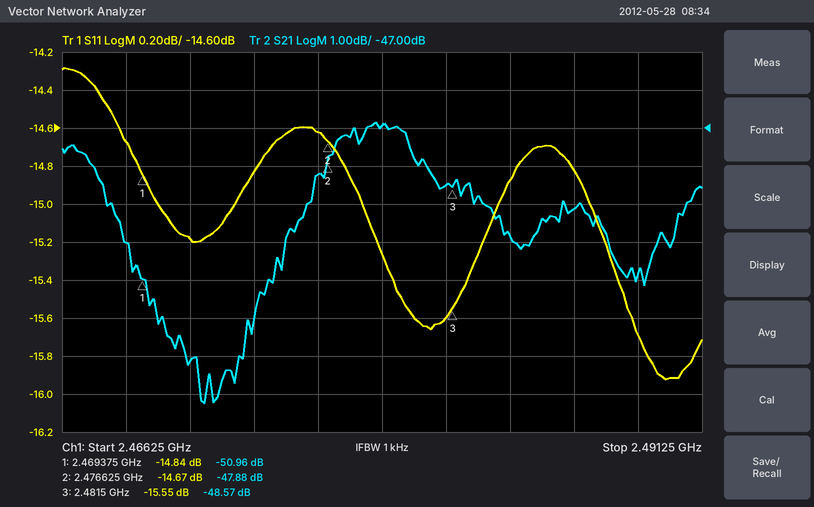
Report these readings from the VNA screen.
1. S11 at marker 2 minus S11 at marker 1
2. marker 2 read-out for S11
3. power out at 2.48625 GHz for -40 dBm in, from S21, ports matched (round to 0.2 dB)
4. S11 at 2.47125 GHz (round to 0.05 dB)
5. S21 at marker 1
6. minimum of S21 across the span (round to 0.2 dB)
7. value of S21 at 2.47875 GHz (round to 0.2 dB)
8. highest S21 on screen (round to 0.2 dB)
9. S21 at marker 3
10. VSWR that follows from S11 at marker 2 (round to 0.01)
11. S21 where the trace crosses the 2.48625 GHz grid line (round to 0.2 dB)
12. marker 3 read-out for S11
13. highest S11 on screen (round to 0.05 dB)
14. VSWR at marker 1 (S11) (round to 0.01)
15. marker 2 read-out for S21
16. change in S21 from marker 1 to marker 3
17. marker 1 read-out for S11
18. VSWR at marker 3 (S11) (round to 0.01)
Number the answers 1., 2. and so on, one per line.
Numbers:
1. 0.17 dB
2. -14.67 dB
3. -89.2 dBm
4. -15.20 dB
5. -50.96 dB
6. -54.2 dB
7. -47.0 dB
8. -46.8 dB
9. -48.57 dB
10. 1.45
11. -49.2 dB
12. -15.55 dB
13. -14.30 dB
14. 1.44
15. -47.88 dB
16. 2.39 dB
17. -14.84 dB
18. 1.40
